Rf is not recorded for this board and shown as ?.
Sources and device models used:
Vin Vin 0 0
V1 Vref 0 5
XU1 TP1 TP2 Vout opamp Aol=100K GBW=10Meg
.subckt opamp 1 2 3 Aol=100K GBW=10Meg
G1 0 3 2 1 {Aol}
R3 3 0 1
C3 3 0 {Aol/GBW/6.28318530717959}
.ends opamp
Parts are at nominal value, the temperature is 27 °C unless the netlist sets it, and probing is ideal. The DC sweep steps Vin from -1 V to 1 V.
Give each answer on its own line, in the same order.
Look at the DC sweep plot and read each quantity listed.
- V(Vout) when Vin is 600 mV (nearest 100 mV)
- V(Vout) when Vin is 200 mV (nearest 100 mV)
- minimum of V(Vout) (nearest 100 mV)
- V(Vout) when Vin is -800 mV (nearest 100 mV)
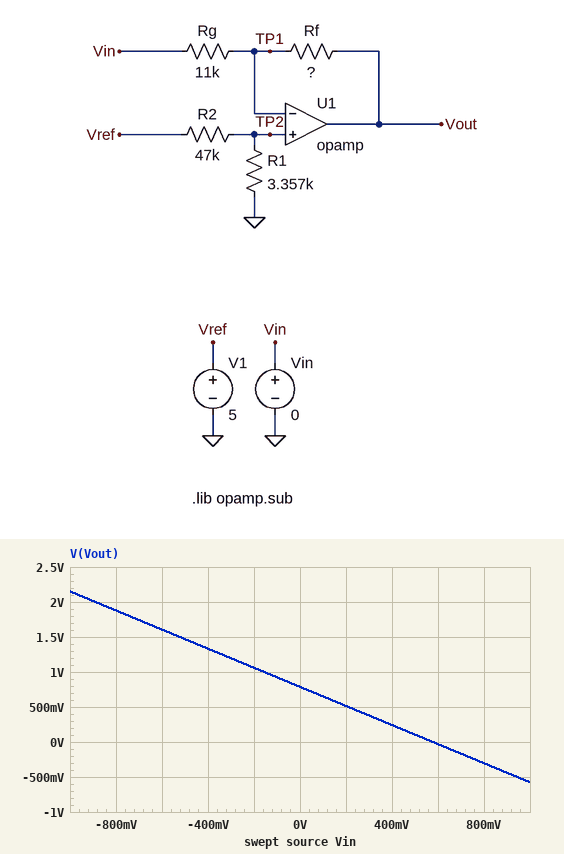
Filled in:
0 V
500 mV
-600 mV
1.9 V
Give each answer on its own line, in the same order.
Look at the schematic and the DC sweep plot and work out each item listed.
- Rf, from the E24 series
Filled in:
15 kΩ
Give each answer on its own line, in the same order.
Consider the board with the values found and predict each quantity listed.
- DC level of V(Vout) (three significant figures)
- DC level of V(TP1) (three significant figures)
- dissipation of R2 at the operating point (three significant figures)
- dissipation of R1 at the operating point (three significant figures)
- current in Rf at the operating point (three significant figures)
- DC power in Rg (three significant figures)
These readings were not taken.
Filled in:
788 mV
333 mV
463 µW
33.1 µW
30.3 µA
10.1 µW
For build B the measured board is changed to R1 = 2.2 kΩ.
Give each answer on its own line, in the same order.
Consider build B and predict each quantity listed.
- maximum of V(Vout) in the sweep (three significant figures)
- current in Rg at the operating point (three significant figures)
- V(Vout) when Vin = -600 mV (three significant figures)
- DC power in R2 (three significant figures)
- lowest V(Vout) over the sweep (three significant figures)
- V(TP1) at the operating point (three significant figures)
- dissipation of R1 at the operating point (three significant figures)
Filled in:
1.89 V
20.3 µA
1.35 V
485 µW
-835 mV
224 mV
22.7 µW
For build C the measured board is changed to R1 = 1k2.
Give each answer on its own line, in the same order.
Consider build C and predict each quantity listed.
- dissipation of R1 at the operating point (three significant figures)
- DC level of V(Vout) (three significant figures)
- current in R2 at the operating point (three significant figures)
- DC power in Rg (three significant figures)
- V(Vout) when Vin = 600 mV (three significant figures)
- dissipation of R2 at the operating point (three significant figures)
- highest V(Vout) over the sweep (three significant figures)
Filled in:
12.9 µW
294 mV
104 µA
1.41 µW
-524 mV
506 µW
1.66 V
